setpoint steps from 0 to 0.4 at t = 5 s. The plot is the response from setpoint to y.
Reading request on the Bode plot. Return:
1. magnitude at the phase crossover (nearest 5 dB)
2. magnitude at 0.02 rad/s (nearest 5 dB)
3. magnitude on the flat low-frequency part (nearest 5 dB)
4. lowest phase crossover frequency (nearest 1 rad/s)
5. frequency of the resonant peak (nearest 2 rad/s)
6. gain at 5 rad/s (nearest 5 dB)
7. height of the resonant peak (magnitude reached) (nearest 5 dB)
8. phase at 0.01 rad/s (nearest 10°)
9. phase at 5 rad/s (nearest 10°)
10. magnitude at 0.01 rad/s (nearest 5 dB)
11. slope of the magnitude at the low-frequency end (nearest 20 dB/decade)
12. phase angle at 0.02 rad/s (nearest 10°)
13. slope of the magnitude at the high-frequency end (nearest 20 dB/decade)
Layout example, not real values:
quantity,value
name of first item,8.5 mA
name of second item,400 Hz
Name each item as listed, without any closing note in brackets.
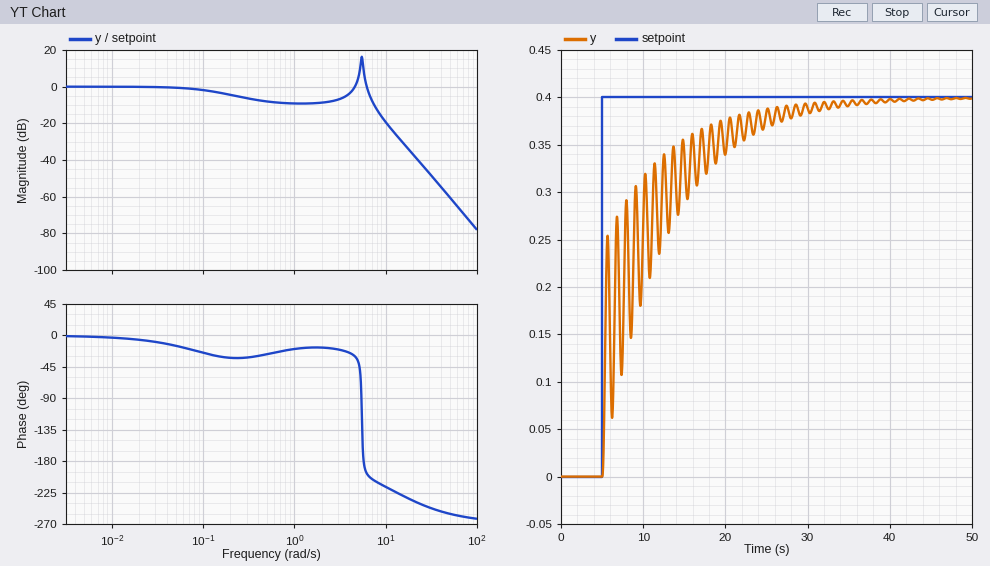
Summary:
quantity,value
magnitude at the phase crossover,10 dB
magnitude at 0.02 rad/s,0 dB
magnitude on the flat low-frequency part,0 dB
lowest phase crossover frequency,6 rad/s
frequency of the resonant peak,6 rad/s
gain at 5 rad/s,5 dB
height of the resonant peak (magnitude reached),15 dB
phase at 0.01 rad/s,0°
phase at 5 rad/s,-40°
magnitude at 0.01 rad/s,0 dB
slope of the magnitude at the low-frequency end,0 dB/decade
phase angle at 0.02 rad/s,-10°
slope of the magnitude at the high-frequency end,-60 dB/decade
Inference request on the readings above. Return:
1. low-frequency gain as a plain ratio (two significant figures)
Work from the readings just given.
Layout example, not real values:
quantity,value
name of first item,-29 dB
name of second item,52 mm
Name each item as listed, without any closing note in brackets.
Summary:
quantity,value
low-frequency gain as a plain ratio,1.0
